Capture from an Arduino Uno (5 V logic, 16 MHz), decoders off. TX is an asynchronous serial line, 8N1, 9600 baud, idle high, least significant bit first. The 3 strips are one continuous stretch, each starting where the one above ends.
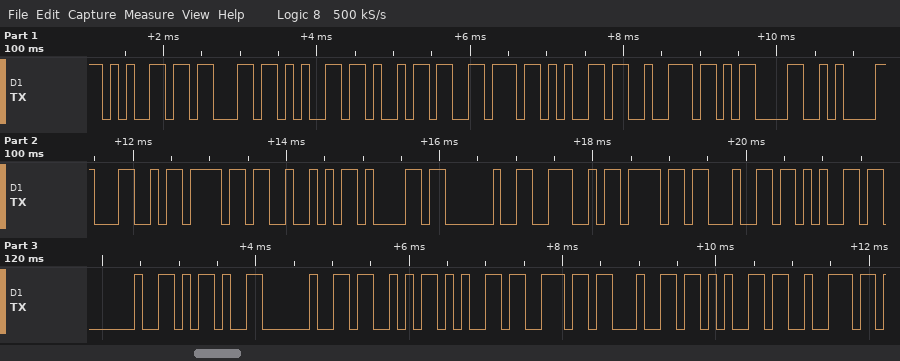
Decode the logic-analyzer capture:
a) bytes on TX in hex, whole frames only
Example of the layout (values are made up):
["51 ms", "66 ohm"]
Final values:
["0x65 0x63 0x65 0x69 0x76 0x65 0x72 0x0D 0x0A 0x4C 0x6F 0x52 0x61 0x20 0x4E 0x6F 0x64 0x65 0x20 0x2D 0x20 0x53 0x65 0x6E 0x64 0x65 0x72"]
